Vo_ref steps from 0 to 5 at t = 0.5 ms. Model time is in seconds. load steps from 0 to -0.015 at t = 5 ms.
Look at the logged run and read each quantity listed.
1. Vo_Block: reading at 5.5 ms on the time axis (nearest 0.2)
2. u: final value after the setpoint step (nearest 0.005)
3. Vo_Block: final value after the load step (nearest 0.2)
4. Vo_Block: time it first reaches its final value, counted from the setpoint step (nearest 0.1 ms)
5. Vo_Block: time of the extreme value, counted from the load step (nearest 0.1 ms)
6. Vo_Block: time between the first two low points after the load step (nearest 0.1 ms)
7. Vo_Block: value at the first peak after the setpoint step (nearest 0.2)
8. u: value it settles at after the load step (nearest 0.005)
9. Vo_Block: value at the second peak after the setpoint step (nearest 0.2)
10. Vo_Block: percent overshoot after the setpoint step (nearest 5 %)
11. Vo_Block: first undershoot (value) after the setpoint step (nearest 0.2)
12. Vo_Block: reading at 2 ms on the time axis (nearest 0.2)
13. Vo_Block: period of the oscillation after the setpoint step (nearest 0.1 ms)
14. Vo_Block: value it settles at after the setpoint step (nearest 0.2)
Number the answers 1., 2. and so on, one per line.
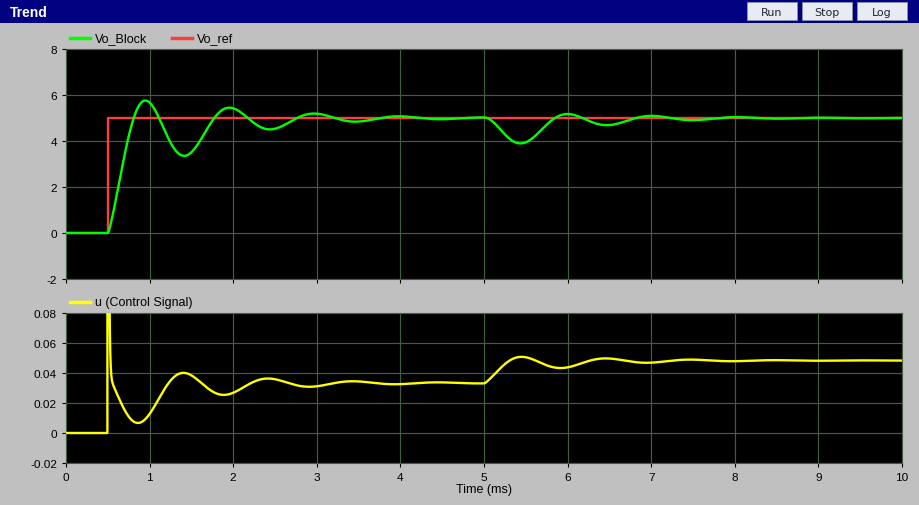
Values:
1. 4.0
2. 0.035
3. 5.0
4. 0.3 ms
5. 0.4 ms
6. 1.0 ms
7. 5.8
8. 0.050
9. 5.4
10. 15 %
11. 3.4
12. 5.4
13. 1.0 ms
14. 5.0
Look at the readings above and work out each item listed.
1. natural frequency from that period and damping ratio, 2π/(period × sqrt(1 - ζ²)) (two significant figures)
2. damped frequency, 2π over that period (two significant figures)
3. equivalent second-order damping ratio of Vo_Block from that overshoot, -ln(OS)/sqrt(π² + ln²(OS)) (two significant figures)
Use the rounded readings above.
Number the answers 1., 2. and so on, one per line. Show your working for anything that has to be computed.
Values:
1. 2π / (1 × sqrt(1 - 0.52²)) = 7.4 rad/ms
2. 2π / 1 = 6.3 rad/ms
3. ln(0.15) = -1.897; 1.897 / sqrt(9.870 + 3.599) = 0.52
